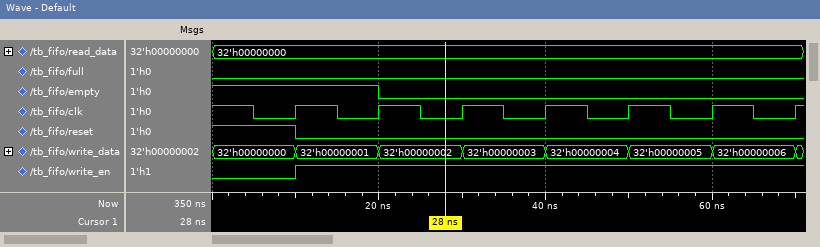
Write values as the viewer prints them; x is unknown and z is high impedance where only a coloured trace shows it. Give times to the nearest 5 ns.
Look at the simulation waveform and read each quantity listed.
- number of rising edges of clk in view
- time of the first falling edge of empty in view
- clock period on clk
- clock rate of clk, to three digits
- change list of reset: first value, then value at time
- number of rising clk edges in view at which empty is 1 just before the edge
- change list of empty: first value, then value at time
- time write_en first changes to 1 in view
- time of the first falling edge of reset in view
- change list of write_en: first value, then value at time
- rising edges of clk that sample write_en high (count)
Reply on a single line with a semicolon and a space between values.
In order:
7; 20 ns; 10 ns; 100 MHz; 1, 0 at 10 ns; 2; 1, 0 at 20 ns; 10 ns; 10 ns; 0, 1 at 10 ns; 6
